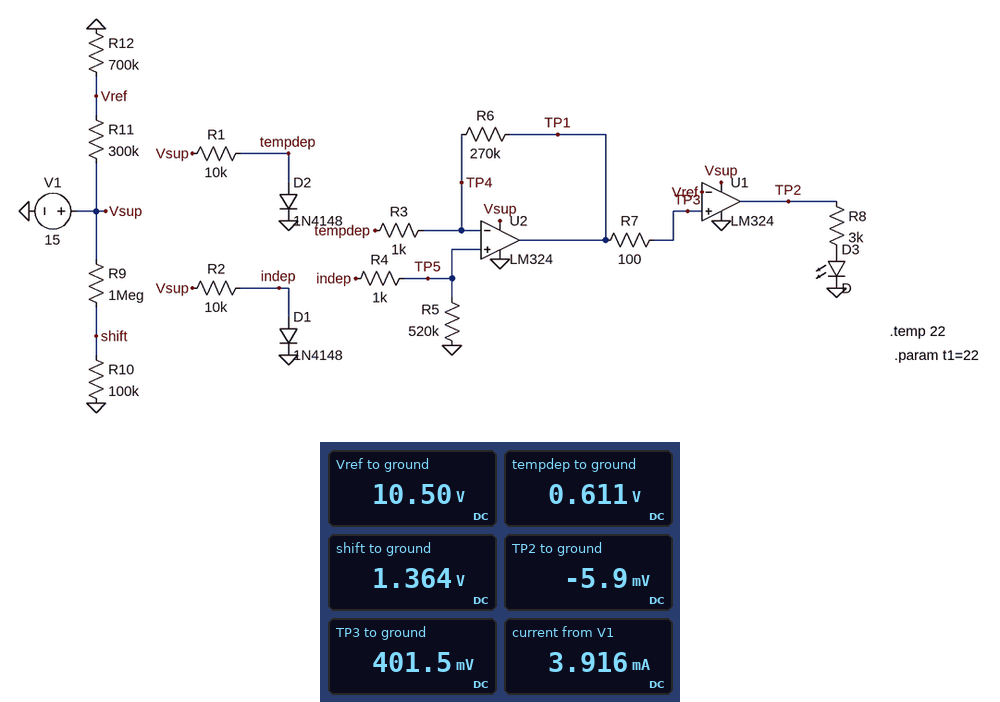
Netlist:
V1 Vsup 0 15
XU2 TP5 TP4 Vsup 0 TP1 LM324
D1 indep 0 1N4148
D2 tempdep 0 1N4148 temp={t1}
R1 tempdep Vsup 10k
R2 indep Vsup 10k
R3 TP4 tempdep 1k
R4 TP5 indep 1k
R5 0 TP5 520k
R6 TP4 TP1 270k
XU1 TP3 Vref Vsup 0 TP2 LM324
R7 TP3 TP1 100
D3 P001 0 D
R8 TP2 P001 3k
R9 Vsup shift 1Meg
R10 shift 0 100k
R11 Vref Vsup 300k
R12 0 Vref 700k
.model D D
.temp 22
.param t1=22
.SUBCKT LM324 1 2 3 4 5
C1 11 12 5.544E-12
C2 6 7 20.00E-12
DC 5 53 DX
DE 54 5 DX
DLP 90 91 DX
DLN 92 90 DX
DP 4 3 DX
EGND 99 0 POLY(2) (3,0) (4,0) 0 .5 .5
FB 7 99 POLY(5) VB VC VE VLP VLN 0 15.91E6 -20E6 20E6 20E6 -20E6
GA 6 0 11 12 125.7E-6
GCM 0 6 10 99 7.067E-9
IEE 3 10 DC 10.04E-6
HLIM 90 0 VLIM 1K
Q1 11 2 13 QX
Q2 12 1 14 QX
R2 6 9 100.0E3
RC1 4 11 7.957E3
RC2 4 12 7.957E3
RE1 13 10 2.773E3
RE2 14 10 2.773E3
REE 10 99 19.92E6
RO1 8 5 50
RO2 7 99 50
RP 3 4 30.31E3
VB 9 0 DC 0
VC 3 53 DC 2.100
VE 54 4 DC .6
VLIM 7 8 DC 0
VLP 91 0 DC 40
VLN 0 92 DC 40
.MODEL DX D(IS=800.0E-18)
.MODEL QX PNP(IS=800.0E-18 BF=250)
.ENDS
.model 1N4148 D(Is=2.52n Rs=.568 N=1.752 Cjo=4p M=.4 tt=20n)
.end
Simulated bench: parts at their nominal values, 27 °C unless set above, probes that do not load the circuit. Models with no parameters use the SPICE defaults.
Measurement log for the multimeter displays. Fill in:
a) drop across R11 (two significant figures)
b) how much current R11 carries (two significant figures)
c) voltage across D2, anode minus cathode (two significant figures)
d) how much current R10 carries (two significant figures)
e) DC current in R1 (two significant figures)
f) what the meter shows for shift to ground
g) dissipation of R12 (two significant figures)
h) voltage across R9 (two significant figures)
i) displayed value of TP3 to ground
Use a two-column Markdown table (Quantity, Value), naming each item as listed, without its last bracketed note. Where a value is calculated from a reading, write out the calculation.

| Quantity | Value |
|---|---|
| drop across R11 | 15 V - 10.5 V = 4.5 V |
| how much current R11 carries | (15 V - 10.5 V) / 300 kΩ = 15 µA |
| voltage across D2, anode minus cathode | 611 mV = 610 mV |
| how much current R10 carries | (1.364 V) / 100 kΩ = 14 µA |
| DC current in R1 | (15 V - 611 mV) / 10 kΩ = 1.4 mA |
| what the meter shows for shift to ground | 1.364 V |
| dissipation of R12 | (10.5 V)^2 / 700 kΩ = 160 µW |
| voltage across R9 | 15 V - 1.364 V = 14 V |
| displayed value of TP3 to ground | 401.5 mV |
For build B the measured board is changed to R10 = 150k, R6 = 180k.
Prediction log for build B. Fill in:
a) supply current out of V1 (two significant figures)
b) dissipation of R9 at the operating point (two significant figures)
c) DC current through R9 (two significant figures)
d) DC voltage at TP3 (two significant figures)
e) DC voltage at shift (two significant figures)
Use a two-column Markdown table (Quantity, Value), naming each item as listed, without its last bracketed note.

| Quantity | Value |
|---|---|
| supply current out of V1 | 3.9 mA |
| dissipation of R9 at the operating point | 170 µW |
| DC current through R9 | 13 µA |
| DC voltage at TP3 | 470 mV |
| DC voltage at shift | 2.0 V |
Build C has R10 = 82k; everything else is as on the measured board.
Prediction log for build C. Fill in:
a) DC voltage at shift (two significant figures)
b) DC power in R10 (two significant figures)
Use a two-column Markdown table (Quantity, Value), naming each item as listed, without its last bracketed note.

| Quantity | Value |
|---|---|
| DC voltage at shift | 1.1 V |
| DC power in R10 | 16 µW |
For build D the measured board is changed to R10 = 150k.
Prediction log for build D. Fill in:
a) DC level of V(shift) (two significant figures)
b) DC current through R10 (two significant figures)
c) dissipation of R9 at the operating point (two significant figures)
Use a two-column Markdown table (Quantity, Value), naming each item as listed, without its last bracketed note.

| Quantity | Value |
|---|---|
| DC level of V(shift) | 2.0 V |
| DC current through R10 | 13 µA |
| dissipation of R9 at the operating point | 170 µW |
